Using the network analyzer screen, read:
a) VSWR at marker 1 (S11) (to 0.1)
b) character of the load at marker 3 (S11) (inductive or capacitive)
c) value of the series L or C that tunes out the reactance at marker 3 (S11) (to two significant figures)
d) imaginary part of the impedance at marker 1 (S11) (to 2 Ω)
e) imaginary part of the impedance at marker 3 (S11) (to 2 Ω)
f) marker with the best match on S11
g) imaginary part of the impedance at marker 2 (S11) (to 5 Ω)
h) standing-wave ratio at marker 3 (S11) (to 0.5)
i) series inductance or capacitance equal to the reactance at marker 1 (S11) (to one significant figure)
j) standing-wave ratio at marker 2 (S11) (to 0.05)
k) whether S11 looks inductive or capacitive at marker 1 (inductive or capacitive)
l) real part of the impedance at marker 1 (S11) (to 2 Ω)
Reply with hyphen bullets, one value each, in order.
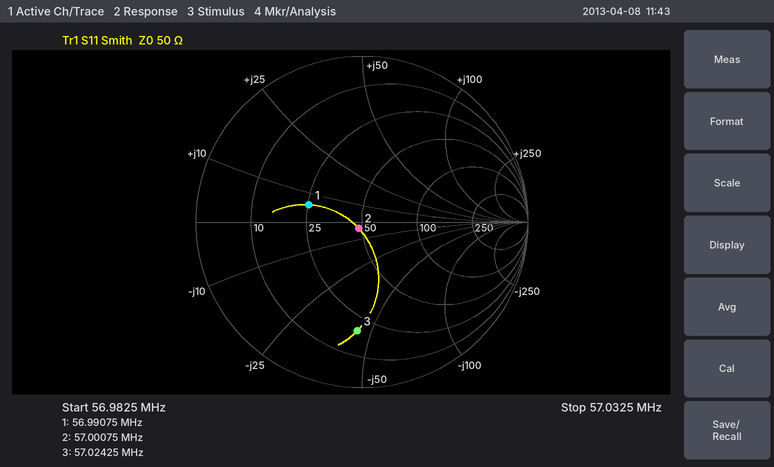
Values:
- 2.0
- capacitive
- 120 nH
- +6 Ω
- -44 Ω
- marker 2
- -5 Ω
- 5.0
- 20 nH
- 1.10
- inductive
- 26 Ω
